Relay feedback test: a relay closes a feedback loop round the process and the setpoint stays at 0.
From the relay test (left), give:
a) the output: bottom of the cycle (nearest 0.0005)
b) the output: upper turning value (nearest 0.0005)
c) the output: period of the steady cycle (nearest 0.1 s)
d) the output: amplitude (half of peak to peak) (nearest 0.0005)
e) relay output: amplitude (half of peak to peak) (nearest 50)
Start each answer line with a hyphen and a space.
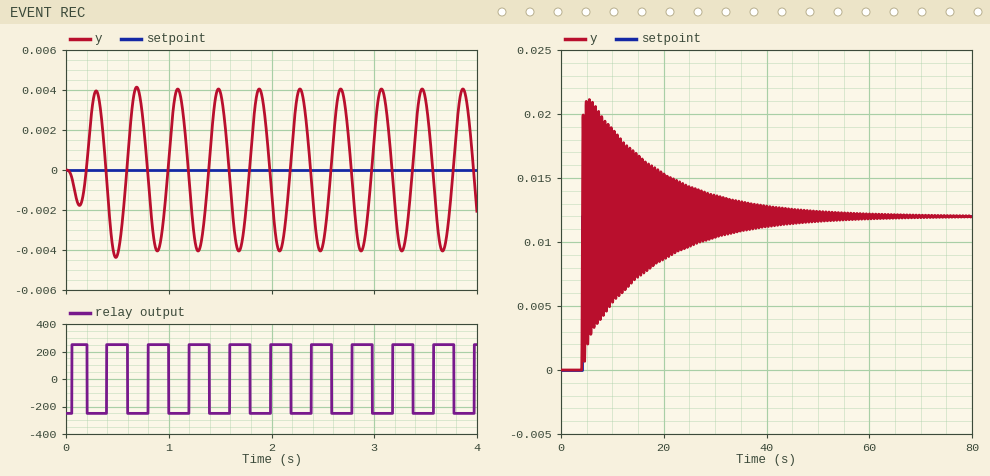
- -0.0040
- 0.0040
- 0.4 s
- 0.0040
- 250
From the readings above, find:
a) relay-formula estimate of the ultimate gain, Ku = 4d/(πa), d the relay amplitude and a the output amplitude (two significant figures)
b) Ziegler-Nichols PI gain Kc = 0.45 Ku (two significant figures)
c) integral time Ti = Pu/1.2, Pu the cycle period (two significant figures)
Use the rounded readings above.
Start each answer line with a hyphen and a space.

- 80000
- 36000
- 0.33 s
